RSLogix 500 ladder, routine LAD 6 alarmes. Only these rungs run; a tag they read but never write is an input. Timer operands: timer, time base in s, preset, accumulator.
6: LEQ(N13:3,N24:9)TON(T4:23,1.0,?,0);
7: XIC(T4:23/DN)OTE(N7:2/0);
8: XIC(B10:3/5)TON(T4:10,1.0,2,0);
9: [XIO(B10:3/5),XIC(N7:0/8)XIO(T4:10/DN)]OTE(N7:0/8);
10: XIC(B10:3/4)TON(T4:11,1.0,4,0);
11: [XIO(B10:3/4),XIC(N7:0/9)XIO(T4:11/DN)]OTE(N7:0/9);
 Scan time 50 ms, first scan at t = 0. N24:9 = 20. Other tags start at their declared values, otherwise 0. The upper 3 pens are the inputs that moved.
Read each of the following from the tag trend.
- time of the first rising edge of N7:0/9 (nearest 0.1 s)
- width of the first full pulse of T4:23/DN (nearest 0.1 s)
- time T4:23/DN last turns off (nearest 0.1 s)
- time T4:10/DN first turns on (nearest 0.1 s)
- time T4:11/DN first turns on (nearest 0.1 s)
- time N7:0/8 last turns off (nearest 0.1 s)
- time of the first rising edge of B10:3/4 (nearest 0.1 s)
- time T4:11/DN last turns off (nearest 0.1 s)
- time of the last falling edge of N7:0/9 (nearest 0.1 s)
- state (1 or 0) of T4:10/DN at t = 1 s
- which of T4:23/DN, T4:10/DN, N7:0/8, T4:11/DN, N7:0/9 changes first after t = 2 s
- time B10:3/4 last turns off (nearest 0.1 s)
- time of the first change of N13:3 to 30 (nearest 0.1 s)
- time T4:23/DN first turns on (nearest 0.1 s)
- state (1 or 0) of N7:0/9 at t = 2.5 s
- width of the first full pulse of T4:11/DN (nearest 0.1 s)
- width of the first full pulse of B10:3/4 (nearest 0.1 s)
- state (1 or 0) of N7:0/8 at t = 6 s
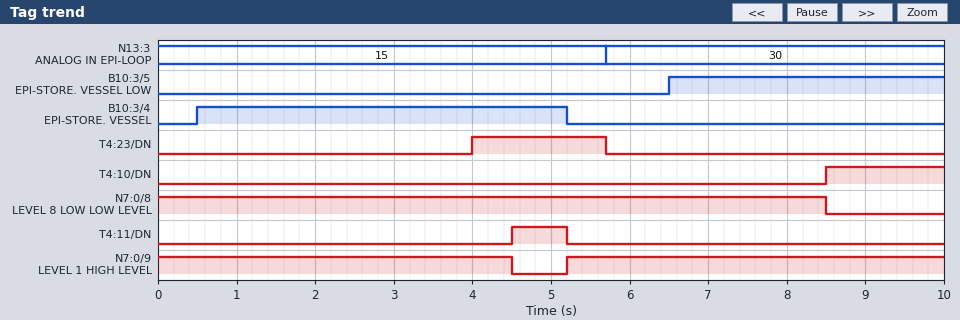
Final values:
5.2 s
1.7 s
5.7 s
8.5 s
4.5 s
8.5 s
0.5 s
5.2 s
4.5 s
0
T4:23/DN
5.2 s
5.7 s
4.0 s
1
0.7 s
4.7 s
1
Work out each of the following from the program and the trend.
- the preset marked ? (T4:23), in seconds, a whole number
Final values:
4 s
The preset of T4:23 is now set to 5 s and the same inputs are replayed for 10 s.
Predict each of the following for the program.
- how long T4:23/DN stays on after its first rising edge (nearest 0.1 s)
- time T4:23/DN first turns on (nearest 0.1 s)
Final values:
0.7 s
5.0 s
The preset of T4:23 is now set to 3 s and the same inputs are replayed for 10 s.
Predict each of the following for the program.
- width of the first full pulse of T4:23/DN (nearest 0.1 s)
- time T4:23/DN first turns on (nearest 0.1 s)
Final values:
2.7 s
3.0 s
